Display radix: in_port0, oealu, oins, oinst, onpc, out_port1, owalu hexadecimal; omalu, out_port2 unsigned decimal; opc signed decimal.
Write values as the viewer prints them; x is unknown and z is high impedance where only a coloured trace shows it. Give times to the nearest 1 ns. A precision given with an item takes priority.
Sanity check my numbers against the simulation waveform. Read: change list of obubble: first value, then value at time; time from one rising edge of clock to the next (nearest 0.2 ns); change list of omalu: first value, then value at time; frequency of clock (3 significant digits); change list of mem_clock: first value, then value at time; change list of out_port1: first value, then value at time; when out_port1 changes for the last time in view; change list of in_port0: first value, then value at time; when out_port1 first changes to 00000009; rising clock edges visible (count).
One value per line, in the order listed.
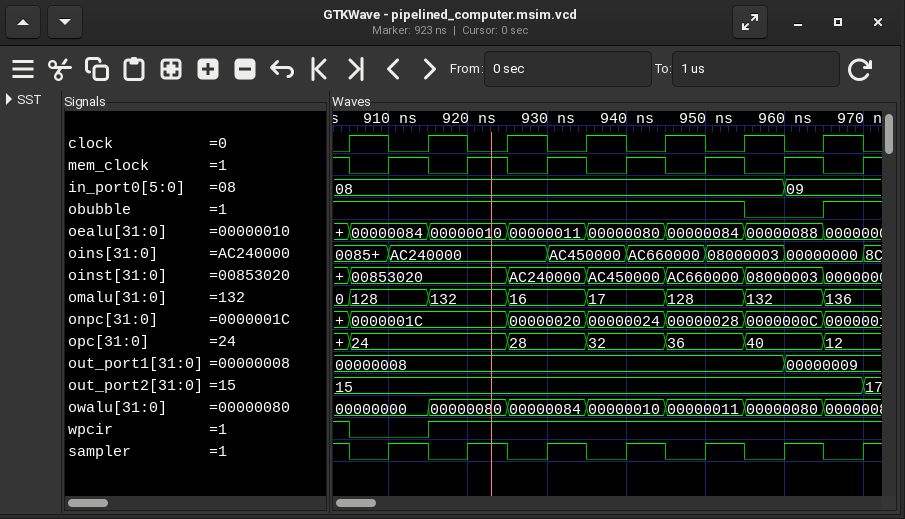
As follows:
1, 0 at 955 ns, 1 at 965 ns
10 ns
0, 128 at 905 ns, 132 at 915 ns, 16 at 925 ns, 17 at 935 ns, 128 at 945 ns, 132 at 955 ns, 136 at 965 ns
100 MHz
1, 0 at 905 ns, 1 at 910 ns, 0 at 915 ns, 1 at 920 ns, 0 at 925 ns, 1 at 930 ns, 0 at 935 ns, 1 at 940 ns, 0 at 945 ns, 1 at 950 ns, 0 at 955 ns, 1 at 960 ns, 0 at 965 ns, 1 at 970 ns
00000008, 00000009 at 960 ns
960 ns
08, 09 at 960 ns
960 ns
7
